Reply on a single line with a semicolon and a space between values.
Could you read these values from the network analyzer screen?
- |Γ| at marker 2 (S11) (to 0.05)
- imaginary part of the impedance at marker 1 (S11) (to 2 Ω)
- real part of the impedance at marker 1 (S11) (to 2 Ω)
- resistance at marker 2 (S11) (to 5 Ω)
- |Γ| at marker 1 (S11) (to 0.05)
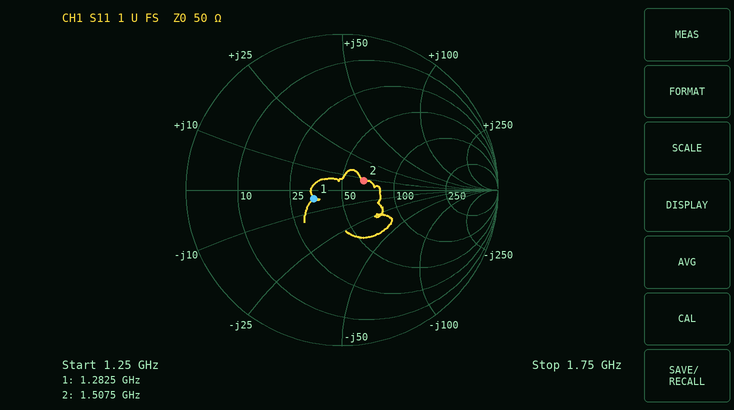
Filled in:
0.15; -4 Ω; 34 Ω; 65 Ω; 0.20
